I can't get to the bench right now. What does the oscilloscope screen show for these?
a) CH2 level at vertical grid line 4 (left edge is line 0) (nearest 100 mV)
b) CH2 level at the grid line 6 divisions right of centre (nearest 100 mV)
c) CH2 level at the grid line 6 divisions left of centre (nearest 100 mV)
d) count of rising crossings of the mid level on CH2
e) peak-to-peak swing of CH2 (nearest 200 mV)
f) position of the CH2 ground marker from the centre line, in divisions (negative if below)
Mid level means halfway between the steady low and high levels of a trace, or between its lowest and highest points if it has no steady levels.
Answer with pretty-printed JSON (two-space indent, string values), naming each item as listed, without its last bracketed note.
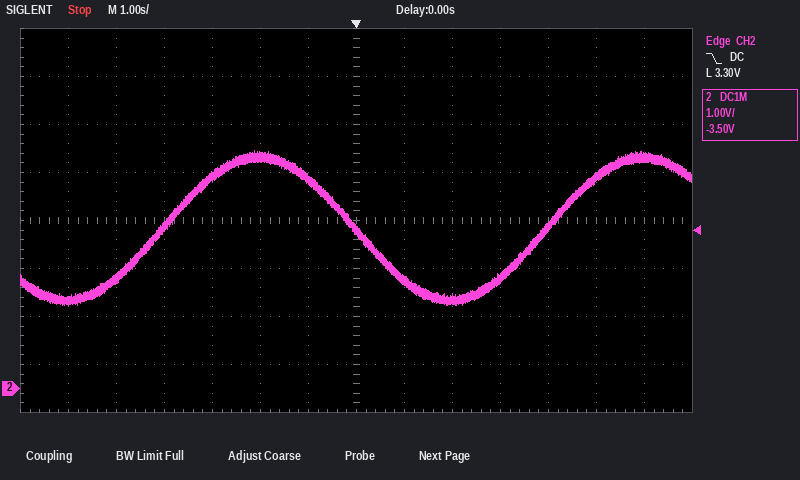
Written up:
{
  "CH2 level at vertical grid line 4 (left edge is line 0)": "4.4 V",
  "CH2 level at the grid line 6 divisions right of centre": "4.8 V",
  "CH2 level at the grid line 6 divisions left of centre": "1.8 V",
  "count of rising crossings of the mid level on CH2": "2",
  "peak-to-peak swing of CH2": "3.2 V",
  "position of the CH2 ground marker from the centre line, in divisions": "-3.5 div"
}
